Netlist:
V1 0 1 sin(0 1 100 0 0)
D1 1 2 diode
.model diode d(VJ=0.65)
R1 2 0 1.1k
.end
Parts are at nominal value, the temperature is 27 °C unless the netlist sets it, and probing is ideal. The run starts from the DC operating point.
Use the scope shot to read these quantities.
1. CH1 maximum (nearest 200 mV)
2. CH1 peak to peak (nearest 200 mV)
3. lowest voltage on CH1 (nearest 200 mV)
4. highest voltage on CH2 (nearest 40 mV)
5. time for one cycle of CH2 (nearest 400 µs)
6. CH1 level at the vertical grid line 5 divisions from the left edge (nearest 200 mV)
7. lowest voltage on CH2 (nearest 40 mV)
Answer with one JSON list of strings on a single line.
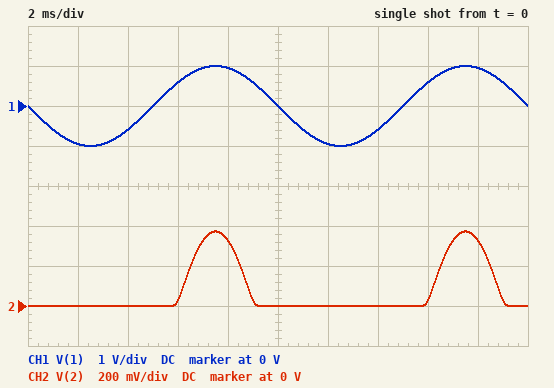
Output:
["1.0 V", "2.0 V", "-1.0 V", "360 mV", "10.0 ms", "0 V", "0 V"]
